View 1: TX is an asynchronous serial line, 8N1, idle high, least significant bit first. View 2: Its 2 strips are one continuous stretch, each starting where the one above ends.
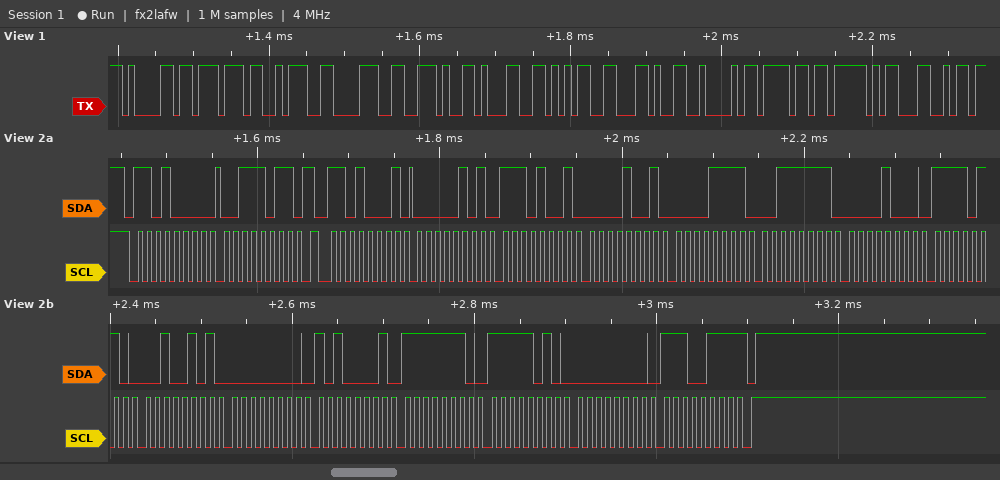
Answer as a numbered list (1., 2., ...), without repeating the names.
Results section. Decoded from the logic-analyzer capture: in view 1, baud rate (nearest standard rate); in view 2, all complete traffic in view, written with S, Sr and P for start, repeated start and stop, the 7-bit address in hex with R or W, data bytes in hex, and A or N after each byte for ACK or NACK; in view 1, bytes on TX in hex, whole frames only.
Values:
1. 115200 baud
2. S 68W A 3B A Sr 68R A 05 A E9 A 09 A 0F A 3F A 08 A F6 A 25 A 00 A A1 A FE A FA A 00 A E7 N P
3. 61 77 3A 38 2E 31 35 2C 42 6F 5F 4C
